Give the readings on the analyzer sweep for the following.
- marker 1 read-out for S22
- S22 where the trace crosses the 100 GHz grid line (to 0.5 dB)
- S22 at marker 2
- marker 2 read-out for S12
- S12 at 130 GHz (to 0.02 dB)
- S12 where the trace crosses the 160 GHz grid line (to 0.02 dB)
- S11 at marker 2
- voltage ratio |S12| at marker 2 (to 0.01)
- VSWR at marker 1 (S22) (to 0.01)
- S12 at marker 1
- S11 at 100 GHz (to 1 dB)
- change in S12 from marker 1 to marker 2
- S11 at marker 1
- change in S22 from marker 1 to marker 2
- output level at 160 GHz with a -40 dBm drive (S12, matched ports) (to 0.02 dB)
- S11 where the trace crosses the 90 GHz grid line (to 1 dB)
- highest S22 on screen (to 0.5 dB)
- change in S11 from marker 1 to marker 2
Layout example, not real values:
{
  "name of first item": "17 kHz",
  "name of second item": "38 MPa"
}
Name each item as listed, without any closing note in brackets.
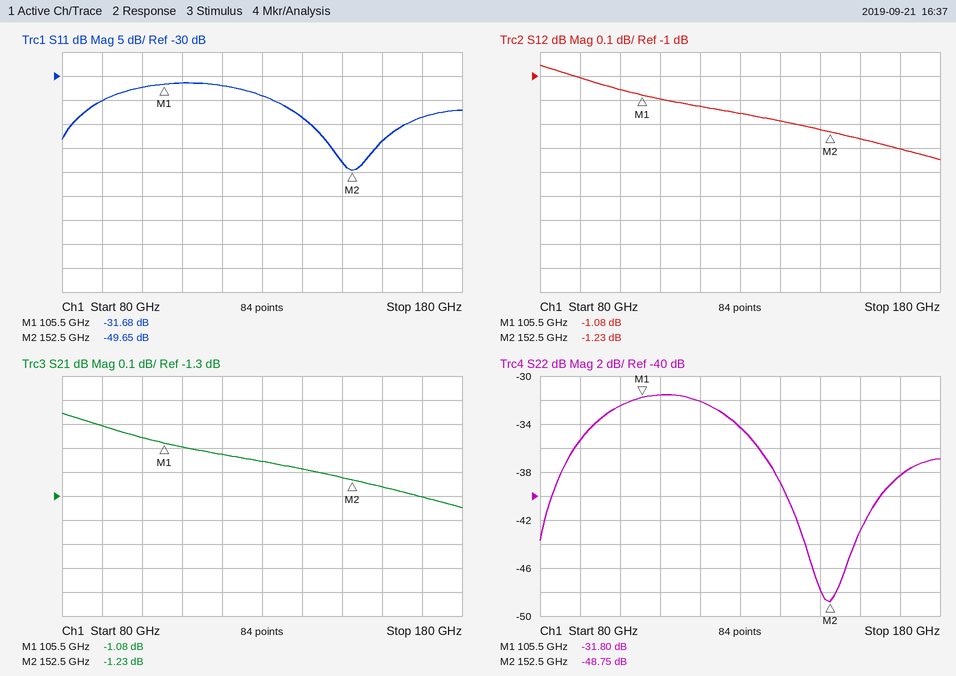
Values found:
{
  "marker 1 read-out for S22": "-31.80 dB",
  "S22 where the trace crosses the 100 GHz grid line": "-32.5 dB",
  "S22 at marker 2": "-48.75 dB",
  "marker 2 read-out for S12": "-1.23 dB",
  "S12 at 130 GHz": "-1.16 dB",
  "S12 where the trace crosses the 160 GHz grid line": "-1.26 dB",
  "S11 at marker 2": "-49.65 dB",
  "voltage ratio |S12| at marker 2": "0.87",
  "VSWR at marker 1 (S22)": "1.05",
  "S12 at marker 1": "-1.08 dB",
  "S11 at 100 GHz": "-32 dB",
  "change in S12 from marker 1 to marker 2": "-0.15 dB",
  "S11 at marker 1": "-31.68 dB",
  "change in S22 from marker 1 to marker 2": "-16.95 dB",
  "output level at 160 GHz with a -40 dBm drive (S12, matched ports)": "-41.26 dBm",
  "S11 where the trace crosses the 90 GHz grid line": "-35 dB",
  "highest S22 on screen": "-31.5 dB",
  "change in S11 from marker 1 to marker 2": "-17.97 dB"
}
